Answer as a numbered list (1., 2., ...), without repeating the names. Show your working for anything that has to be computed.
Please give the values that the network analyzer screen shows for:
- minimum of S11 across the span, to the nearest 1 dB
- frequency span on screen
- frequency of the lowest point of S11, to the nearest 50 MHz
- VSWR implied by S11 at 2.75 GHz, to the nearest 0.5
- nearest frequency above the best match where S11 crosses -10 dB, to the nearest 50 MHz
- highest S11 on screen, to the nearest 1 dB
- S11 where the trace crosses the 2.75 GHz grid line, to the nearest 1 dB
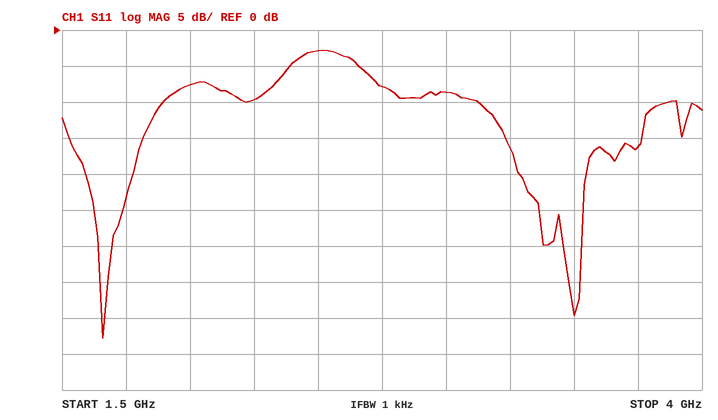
1. -43 dB
2. 2.5 GHz
3. 1.65 GHz
4. |Γ| = 10^(-8/20) = 0.3981; VSWR = (1 + 0.3981)/(1 − 0.3981) ≈ 2.32, so 2.5 to the nearest 0.5
5. 1.90 GHz
6. -3 dB
7. -8 dB
